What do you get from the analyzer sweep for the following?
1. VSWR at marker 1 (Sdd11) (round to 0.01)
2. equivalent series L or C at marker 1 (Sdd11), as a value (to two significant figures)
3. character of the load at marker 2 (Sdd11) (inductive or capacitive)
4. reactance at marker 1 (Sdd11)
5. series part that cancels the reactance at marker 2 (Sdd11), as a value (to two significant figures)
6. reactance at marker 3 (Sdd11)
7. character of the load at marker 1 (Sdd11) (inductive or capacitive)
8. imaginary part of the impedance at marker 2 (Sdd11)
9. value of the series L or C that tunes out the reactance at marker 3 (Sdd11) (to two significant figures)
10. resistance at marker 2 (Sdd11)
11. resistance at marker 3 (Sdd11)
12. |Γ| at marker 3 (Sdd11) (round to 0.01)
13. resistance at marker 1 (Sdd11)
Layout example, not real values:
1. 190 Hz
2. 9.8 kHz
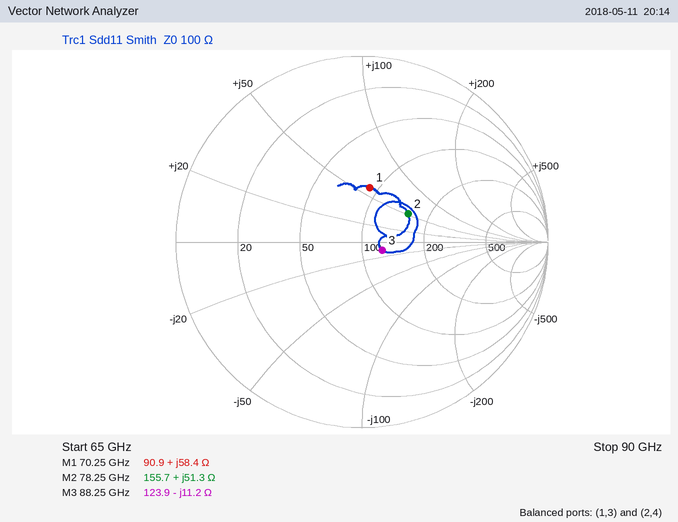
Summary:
1. 1.84
2. 130 pH
3. inductive
4. +58.4 Ω
5. 40 fF
6. -11.2 Ω
7. inductive
8. +51.3 Ω
9. 20 pH
10. 155.7 Ω
11. 123.9 Ω
12. 0.12
13. 90.9 Ω
